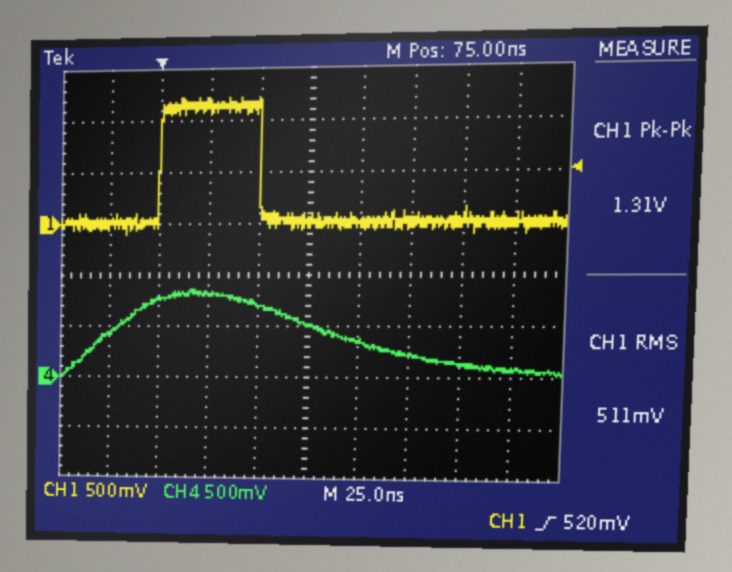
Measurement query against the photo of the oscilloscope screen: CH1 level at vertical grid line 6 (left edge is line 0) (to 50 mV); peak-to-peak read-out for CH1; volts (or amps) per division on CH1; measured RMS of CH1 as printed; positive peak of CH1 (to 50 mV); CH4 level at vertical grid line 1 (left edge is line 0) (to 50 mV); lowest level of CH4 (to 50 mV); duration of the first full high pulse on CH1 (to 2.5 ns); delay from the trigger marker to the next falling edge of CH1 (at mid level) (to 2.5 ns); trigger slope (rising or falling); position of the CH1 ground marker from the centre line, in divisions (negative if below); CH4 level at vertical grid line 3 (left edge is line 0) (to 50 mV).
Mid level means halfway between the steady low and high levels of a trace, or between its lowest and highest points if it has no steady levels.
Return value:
0 mV
1.31 V
500 mV
511 mV
1.20 V
450 mV
0 mV
50.0 ns
50.0 ns
rising
+1.0 div
800 mV
